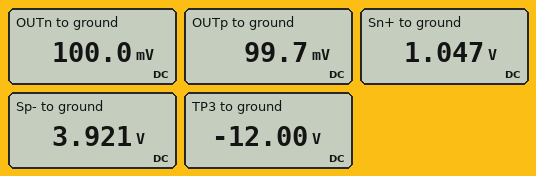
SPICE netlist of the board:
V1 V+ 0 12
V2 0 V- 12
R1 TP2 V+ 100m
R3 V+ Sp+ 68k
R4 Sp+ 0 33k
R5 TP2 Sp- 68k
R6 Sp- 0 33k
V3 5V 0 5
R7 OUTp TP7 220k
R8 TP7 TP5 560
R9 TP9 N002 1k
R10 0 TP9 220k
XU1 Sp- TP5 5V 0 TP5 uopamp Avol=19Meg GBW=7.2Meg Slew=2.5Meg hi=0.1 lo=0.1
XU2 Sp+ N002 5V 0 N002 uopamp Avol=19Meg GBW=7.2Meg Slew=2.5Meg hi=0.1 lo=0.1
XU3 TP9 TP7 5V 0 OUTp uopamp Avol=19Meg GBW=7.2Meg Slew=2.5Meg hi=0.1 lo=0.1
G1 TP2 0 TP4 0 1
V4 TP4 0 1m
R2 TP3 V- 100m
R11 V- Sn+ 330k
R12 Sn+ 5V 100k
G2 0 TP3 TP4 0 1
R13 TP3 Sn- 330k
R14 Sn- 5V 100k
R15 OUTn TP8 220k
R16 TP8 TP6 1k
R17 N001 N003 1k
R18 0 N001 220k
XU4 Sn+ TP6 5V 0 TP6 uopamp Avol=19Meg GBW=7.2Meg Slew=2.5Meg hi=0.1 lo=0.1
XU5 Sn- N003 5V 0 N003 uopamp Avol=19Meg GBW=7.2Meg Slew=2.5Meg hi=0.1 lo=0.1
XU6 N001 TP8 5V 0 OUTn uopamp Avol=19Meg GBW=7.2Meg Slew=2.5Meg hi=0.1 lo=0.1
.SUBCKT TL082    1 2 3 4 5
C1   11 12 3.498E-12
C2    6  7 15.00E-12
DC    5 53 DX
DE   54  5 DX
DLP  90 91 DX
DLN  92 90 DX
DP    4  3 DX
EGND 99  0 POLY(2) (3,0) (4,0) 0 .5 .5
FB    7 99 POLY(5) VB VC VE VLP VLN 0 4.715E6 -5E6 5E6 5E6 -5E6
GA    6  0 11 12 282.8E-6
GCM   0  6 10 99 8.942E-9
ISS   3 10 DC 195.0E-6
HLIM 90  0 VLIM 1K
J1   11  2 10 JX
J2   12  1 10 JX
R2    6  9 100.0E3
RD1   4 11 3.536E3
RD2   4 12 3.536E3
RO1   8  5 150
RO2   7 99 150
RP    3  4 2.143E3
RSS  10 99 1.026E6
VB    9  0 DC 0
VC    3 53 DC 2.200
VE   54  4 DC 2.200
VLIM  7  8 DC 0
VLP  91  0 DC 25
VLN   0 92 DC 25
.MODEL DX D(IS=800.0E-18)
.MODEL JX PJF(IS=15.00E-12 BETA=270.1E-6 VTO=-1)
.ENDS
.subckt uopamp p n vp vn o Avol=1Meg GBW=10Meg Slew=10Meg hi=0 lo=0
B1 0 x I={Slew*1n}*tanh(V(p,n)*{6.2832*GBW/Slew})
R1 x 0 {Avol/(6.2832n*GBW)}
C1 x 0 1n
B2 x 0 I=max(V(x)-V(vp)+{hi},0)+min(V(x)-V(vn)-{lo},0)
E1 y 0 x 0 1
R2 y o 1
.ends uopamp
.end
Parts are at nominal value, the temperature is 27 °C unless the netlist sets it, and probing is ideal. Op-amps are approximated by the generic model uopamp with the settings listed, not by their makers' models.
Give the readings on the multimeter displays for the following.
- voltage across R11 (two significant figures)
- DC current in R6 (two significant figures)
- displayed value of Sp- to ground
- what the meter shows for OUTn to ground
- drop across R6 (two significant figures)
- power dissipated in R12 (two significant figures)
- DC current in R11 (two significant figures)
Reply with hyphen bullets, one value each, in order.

- 13 V
- 120 µA
- 3.921 V
- 100.0 mV
- 3.9 V
- 160 µW
- 40 µA
